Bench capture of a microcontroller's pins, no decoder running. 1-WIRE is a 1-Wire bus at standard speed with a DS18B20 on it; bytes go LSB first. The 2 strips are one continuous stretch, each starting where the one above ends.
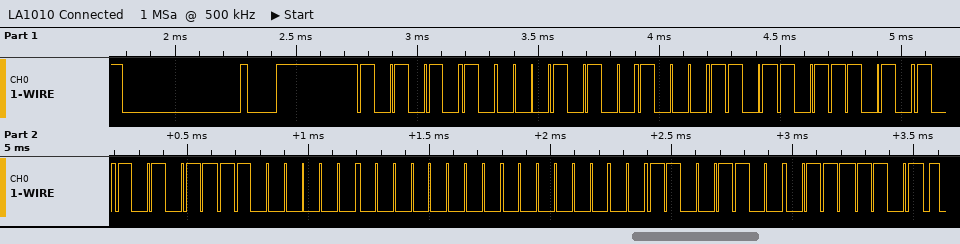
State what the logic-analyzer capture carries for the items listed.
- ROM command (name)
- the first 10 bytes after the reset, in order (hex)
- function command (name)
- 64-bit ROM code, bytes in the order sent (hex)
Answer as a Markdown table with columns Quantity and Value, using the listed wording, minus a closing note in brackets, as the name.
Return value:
| Quantity | Value |
|---|---|
| ROM command | Match ROM |
| the first 10 bytes after the reset, in order | 55 28 B1 5D D5 03 00 00 33 BE |
| function command | Read Scratchpad |
| 64-bit ROM code, bytes in the order sent | 28 B1 5D D5 03 00 00 33 |
